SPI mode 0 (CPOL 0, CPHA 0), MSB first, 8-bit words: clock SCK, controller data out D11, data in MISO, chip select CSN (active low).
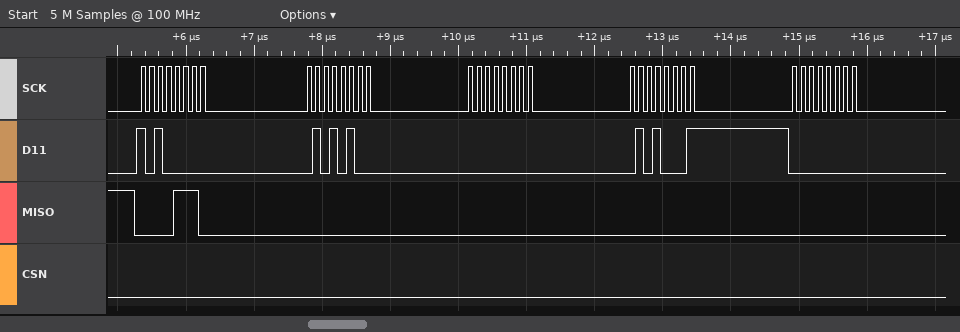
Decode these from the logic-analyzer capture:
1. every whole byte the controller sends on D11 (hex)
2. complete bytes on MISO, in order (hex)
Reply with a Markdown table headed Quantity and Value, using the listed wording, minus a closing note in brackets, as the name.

| Quantity | Value |
|---|---|
| every whole byte the controller sends on D11 | 0xA0 0x54 0x00 0x51 0x00 |
| complete bytes on MISO, in order | 0x0E 0x00 0x00 0x00 0x00 |
